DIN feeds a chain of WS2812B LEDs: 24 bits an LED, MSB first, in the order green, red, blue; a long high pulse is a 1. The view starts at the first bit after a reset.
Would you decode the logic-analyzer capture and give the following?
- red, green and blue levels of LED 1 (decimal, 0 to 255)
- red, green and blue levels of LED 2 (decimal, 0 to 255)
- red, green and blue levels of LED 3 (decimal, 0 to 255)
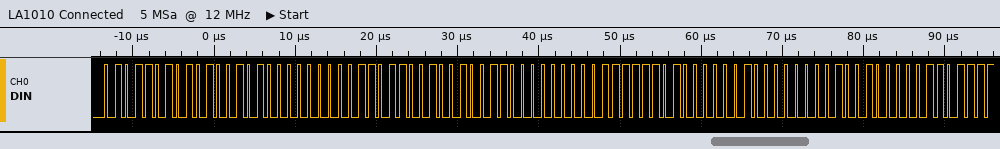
165, 90, 0
147, 108, 0
129, 126, 0
